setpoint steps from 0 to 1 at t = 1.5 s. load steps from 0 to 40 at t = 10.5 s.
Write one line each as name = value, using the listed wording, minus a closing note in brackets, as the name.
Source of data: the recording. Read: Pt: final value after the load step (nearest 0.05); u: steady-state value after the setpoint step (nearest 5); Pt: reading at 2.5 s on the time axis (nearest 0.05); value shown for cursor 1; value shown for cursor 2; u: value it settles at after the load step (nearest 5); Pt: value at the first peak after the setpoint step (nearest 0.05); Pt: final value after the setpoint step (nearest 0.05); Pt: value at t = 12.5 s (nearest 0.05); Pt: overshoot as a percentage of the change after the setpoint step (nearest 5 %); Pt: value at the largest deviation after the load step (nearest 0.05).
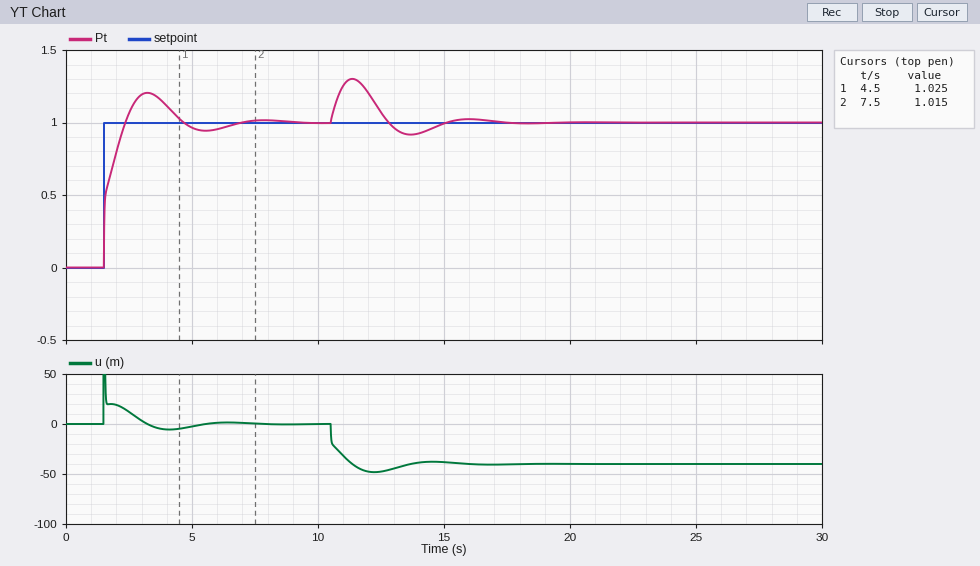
Pt: final value after the load step = 1.00
u: steady-state value after the setpoint step = 0
Pt: reading at 2.5 s on the time axis = 1.05
value shown for cursor 1 = 1.025
value shown for cursor 2 = 1.015
u: value it settles at after the load step = -40
Pt: value at the first peak after the setpoint step = 1.20
Pt: final value after the setpoint step = 1.00
Pt: value at t = 12.5 s = 1.05
Pt: overshoot as a percentage of the change after the setpoint step = 20 %
Pt: value at the largest deviation after the load step = 1.30
